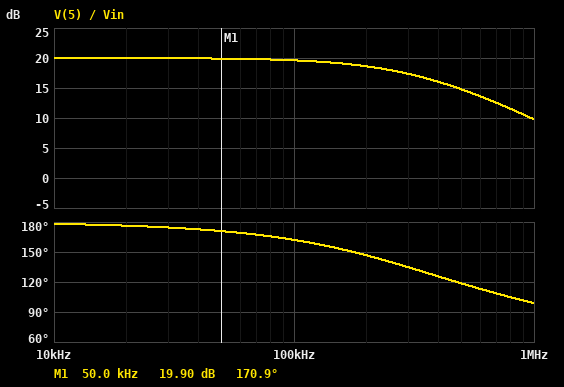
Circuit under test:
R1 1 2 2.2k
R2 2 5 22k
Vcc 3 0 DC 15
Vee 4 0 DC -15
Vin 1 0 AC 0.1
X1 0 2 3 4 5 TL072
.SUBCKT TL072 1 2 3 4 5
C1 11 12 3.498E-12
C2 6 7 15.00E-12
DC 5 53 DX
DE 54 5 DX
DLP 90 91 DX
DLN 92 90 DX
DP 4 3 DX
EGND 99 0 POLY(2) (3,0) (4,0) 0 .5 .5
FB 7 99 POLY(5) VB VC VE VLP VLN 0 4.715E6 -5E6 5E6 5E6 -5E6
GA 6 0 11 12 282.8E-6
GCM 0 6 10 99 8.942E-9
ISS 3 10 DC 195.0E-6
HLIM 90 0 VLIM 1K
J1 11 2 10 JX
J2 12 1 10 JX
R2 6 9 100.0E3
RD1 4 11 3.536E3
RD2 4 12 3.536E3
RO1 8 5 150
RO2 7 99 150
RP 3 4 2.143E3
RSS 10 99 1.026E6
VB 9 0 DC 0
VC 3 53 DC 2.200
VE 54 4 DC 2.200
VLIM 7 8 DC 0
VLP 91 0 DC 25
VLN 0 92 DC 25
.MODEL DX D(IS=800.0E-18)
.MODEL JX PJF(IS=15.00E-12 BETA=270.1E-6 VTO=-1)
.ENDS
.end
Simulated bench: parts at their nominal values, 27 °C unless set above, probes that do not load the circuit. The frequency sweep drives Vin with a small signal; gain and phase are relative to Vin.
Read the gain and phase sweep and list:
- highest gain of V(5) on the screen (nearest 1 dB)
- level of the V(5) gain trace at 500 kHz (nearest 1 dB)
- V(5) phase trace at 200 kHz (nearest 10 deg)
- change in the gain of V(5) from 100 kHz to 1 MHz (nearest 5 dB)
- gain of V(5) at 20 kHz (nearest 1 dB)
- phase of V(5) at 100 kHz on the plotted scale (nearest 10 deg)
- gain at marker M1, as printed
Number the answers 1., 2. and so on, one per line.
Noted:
1. 20 dB
2. 15 dB
3. 150 deg
4. -10 dB
5. 20 dB
6. 160 deg
7. 19.90 dB
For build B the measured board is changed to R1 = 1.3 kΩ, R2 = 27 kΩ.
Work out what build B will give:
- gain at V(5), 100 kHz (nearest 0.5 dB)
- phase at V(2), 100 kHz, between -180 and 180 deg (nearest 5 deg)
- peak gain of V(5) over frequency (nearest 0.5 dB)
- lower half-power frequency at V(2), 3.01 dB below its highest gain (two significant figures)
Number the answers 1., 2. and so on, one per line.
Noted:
1. 25.0 dB
2. 60 deg
3. 26.5 dB
4. 160 kHz
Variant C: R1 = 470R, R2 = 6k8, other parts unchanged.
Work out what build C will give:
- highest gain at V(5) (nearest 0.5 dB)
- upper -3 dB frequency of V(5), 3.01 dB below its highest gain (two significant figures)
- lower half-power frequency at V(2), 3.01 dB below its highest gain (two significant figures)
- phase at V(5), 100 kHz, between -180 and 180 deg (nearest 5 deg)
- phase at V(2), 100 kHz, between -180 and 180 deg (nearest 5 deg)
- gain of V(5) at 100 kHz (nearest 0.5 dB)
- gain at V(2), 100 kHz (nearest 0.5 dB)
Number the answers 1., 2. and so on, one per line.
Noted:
1. 23.0 dB
2. 230 kHz
3. 220 kHz
4. 155 deg
5. 65 deg
6. 22.5 dB
7. -8.0 dB
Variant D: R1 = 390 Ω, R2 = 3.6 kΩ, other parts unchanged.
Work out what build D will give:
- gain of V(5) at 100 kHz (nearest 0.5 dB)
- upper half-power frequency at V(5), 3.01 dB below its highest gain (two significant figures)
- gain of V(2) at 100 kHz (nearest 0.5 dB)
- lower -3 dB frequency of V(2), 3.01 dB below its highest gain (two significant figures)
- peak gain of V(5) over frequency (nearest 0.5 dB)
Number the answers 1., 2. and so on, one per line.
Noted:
1. 19.0 dB
2. 340 kHz
3. -11.5 dB
4. 330 kHz
5. 19.5 dB
